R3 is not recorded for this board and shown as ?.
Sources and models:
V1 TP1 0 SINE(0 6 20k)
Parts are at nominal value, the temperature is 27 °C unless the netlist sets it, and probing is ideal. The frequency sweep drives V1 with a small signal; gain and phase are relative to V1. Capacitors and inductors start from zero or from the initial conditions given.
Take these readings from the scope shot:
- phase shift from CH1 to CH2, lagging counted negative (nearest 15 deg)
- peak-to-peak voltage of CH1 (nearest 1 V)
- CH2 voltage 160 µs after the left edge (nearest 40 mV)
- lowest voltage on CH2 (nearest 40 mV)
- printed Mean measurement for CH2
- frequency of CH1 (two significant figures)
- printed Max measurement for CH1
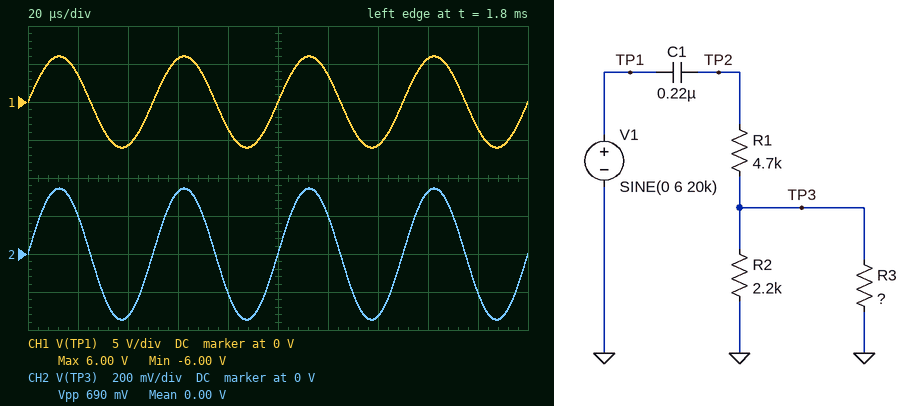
0 deg
12 V
320 mV
-360 mV
0.00 V
20 kHz
6.00 V
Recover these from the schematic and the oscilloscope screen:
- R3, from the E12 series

330 Ω
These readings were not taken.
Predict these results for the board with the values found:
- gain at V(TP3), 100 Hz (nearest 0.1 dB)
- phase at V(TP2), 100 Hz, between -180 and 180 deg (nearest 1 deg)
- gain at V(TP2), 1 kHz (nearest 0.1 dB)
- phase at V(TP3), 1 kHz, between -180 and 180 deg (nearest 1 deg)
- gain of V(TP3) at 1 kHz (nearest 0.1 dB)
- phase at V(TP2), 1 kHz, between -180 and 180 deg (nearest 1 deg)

-29.7 dB
55 deg
-0.1 dB
8 deg
-24.9 dB
8 deg
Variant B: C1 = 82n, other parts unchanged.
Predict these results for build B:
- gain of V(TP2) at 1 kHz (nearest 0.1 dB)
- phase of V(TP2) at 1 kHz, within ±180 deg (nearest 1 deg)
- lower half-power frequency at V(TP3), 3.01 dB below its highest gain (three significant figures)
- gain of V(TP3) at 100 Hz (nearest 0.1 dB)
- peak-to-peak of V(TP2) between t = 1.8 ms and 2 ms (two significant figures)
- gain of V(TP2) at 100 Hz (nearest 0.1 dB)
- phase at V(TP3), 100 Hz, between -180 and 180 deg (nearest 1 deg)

-0.6 dB
21 deg
389 Hz
-36.9 dB
12 V
-12.1 dB
76 deg
